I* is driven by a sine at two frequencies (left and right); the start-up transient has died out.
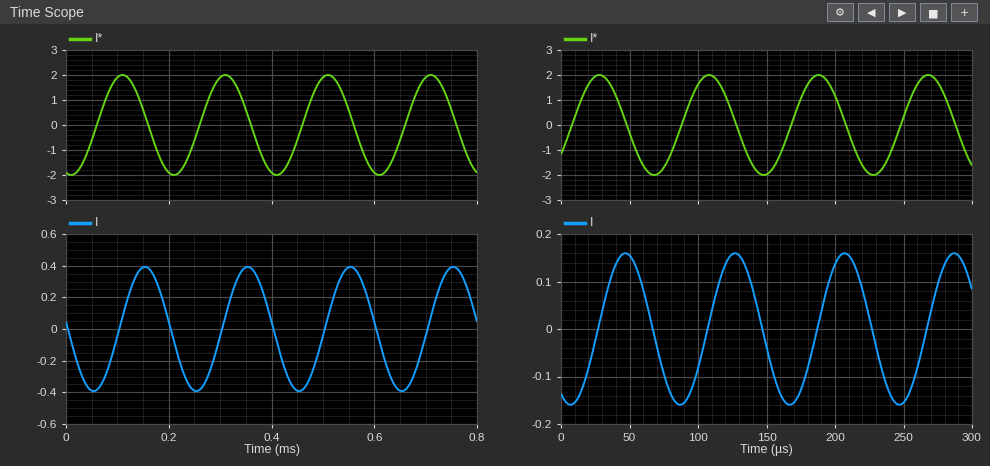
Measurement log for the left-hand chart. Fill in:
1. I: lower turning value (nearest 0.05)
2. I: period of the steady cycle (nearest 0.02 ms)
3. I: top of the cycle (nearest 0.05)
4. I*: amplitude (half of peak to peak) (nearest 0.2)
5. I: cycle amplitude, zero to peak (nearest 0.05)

-0.40
0.20 ms
0.40
2.0
0.40
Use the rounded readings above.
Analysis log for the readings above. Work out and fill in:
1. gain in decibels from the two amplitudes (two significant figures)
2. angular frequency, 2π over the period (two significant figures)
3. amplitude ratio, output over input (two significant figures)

-14 dB
31 rad/ms
0.20
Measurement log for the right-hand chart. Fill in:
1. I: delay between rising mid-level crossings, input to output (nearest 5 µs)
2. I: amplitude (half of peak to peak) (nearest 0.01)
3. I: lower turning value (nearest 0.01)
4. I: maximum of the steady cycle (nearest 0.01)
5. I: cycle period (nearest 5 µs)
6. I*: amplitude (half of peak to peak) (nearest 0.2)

20 µs
0.16
-0.16
0.16
80 µs
2.0
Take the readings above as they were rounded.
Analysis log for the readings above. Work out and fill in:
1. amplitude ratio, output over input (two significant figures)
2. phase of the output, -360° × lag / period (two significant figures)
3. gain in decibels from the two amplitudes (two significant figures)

0.080
-90°
-22 dB
